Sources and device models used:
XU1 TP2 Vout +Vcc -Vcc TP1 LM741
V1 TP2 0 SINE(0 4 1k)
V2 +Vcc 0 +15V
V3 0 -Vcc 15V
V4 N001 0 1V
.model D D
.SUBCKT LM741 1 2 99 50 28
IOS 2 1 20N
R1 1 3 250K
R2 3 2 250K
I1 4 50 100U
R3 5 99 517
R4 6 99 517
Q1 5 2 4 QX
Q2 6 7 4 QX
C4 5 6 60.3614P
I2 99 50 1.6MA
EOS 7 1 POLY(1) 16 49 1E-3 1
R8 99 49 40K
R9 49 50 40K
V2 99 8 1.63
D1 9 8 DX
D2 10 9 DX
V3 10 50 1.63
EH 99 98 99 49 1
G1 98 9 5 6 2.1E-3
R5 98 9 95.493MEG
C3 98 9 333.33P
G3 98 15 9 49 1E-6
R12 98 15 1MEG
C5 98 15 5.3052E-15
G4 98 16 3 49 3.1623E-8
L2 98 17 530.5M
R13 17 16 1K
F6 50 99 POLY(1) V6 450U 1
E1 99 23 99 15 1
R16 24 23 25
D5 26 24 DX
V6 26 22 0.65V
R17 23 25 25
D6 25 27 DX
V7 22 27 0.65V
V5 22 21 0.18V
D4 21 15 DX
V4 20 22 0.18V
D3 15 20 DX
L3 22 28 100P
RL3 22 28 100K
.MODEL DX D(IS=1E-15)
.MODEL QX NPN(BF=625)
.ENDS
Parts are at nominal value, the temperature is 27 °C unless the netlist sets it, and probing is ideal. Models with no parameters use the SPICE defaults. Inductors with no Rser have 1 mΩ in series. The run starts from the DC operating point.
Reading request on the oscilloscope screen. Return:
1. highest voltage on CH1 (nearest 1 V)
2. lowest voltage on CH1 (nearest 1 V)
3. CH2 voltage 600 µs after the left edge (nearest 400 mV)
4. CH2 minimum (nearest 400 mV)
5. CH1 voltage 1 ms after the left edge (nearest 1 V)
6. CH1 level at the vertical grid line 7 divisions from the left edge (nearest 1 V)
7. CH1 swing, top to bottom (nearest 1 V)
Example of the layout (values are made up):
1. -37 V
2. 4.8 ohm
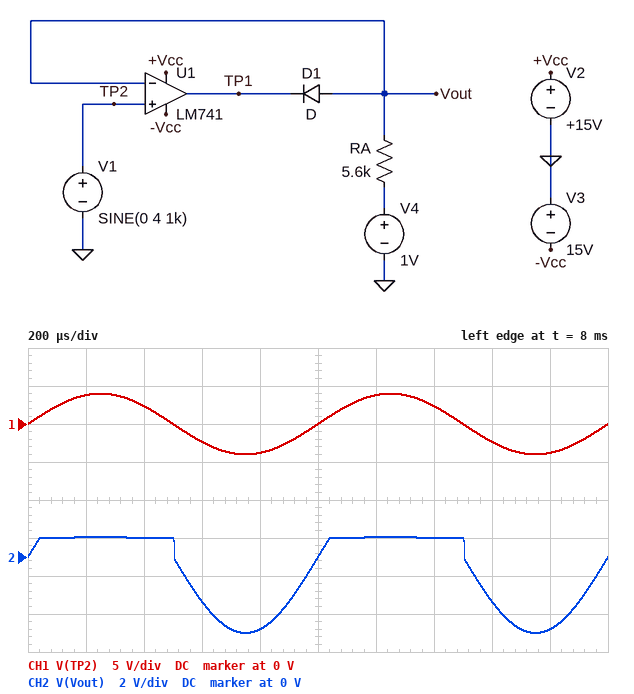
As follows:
1. 4 V
2. -4 V
3. -2.4 V
4. -4.0 V
5. 0 V
6. 2 V
7. 8 V
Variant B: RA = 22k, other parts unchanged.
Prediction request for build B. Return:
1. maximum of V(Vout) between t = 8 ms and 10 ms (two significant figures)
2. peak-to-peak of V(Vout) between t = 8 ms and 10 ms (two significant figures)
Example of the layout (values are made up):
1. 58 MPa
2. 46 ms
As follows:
1. 1.1 V
2. 5.1 V
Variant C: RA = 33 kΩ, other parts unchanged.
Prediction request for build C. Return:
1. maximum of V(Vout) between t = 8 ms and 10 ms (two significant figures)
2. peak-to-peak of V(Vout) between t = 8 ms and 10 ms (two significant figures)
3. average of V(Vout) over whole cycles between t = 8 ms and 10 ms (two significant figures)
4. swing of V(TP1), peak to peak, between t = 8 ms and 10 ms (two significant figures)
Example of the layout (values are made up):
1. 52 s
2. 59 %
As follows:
1. 1.2 V
2. 5.2 V
3. -740 mV
4. 19 V
